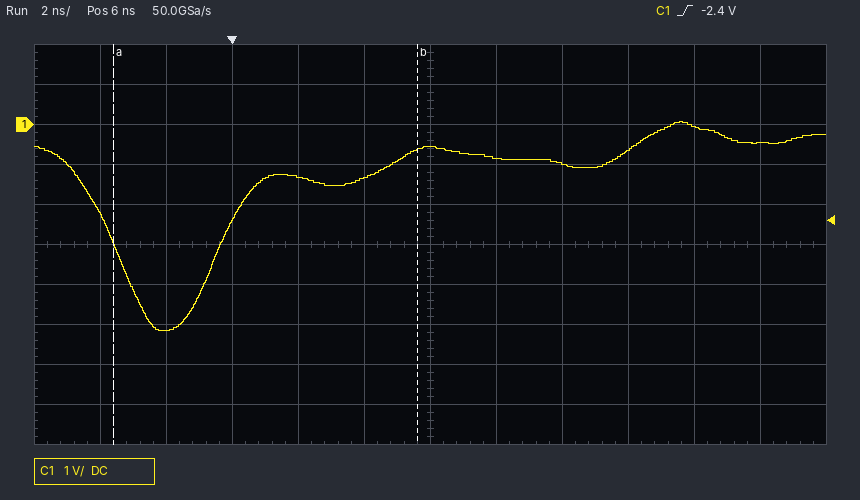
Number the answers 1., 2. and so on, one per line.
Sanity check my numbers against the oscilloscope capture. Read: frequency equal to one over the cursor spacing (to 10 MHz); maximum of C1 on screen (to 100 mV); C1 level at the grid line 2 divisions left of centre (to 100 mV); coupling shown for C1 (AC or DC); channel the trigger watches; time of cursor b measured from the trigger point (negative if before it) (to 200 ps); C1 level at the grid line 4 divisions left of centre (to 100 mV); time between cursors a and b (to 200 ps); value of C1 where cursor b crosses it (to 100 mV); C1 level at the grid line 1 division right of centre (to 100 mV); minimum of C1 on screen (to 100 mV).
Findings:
1. 110 MHz
2. 100 mV
3. -1.3 V
4. DC
5. C1
6. +5.6 ns
7. -5.2 V
8. 9.2 ns
9. -600 mV
10. -800 mV
11. -5.2 V
